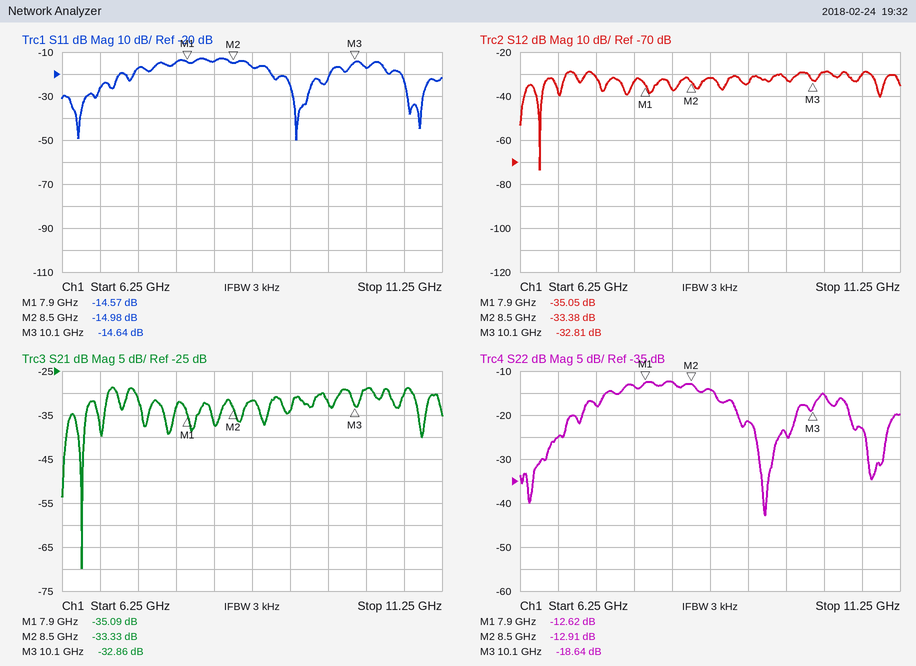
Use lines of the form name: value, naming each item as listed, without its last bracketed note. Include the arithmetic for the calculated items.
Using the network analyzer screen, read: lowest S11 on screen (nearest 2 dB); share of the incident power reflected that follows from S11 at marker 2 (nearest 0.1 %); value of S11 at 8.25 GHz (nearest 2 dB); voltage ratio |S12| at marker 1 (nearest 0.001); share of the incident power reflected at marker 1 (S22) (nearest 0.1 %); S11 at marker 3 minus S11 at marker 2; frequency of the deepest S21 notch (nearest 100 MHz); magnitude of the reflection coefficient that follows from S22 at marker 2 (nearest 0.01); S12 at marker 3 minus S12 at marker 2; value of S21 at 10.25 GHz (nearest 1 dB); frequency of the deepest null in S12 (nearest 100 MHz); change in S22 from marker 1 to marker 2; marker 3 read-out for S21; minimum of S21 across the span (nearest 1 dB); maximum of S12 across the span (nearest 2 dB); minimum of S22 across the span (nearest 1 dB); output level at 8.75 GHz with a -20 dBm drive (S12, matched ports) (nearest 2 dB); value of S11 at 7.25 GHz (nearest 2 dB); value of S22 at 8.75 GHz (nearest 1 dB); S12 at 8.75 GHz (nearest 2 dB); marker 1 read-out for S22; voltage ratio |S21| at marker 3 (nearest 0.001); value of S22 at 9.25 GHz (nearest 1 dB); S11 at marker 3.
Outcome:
lowest S11 on screen: -50 dB
share of the incident power reflected that follows from S11 at marker 2: 10^(-14.98/10) ≈ 3.2 %
value of S11 at 8.25 GHz: -14 dB
voltage ratio |S12| at marker 1: 10^(-35.05/20) ≈ 0.018
share of the incident power reflected at marker 1 (S22): 10^(-12.62/10) ≈ 5.5 %
S11 at marker 3 minus S11 at marker 2: -14.64 − (-14.98) = 0.34 dB
frequency of the deepest S21 notch: 6.5 GHz
magnitude of the reflection coefficient that follows from S22 at marker 2: 10^(-12.91/20) ≈ 0.23
S12 at marker 3 minus S12 at marker 2: -32.81 − (-33.38) = 0.57 dB
value of S21 at 10.25 GHz: -29 dB
frequency of the deepest null in S12: 6.5 GHz
change in S22 from marker 1 to marker 2: -12.91 − (-12.62) = -0.29 dB
marker 3 read-out for S21: -32.86 dB
minimum of S21 across the span: -70 dB
maximum of S12 across the span: -28 dB
minimum of S22 across the span: -43 dB
output level at 8.75 GHz with a -20 dBm drive (S12, matched ports): -20 dBm + (-32 dB) = -52 dBm
value of S11 at 7.25 GHz: -18 dB
value of S22 at 8.75 GHz: -14 dB
S12 at 8.75 GHz: -32 dB
marker 1 read-out for S22: -12.62 dB
voltage ratio |S21| at marker 3: 10^(-32.86/20) ≈ 0.023
value of S22 at 9.25 GHz: -21 dB
S11 at marker 3: -14.64 dB
